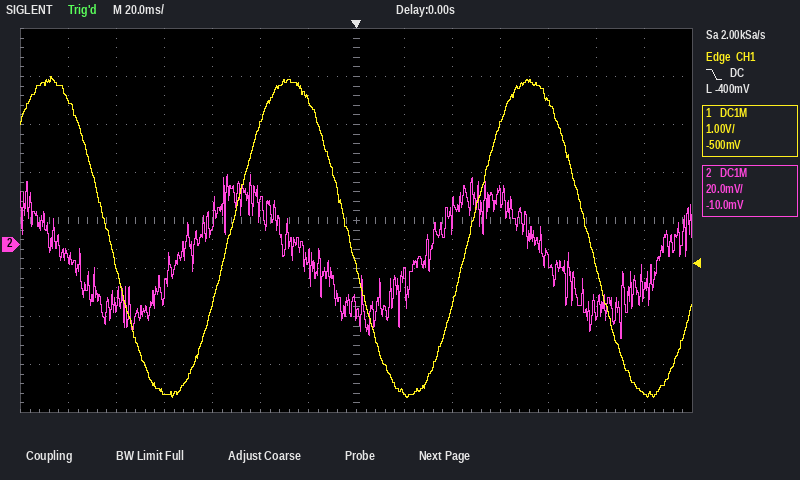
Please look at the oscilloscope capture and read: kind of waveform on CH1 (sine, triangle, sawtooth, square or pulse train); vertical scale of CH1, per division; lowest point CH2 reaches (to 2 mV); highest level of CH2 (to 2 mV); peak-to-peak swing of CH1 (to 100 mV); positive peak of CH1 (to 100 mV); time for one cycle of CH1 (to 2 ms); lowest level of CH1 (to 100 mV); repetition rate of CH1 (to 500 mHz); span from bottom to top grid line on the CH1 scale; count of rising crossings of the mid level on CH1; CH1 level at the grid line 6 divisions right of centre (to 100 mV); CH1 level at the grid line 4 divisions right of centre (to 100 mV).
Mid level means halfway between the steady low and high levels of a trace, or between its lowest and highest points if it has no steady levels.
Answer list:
sine
1 V
-40 mV
30 mV
6.7 V
3.5 V
100 ms
-3.2 V
10.0 Hz
8 V
2
-3.1 V
3.0 V
